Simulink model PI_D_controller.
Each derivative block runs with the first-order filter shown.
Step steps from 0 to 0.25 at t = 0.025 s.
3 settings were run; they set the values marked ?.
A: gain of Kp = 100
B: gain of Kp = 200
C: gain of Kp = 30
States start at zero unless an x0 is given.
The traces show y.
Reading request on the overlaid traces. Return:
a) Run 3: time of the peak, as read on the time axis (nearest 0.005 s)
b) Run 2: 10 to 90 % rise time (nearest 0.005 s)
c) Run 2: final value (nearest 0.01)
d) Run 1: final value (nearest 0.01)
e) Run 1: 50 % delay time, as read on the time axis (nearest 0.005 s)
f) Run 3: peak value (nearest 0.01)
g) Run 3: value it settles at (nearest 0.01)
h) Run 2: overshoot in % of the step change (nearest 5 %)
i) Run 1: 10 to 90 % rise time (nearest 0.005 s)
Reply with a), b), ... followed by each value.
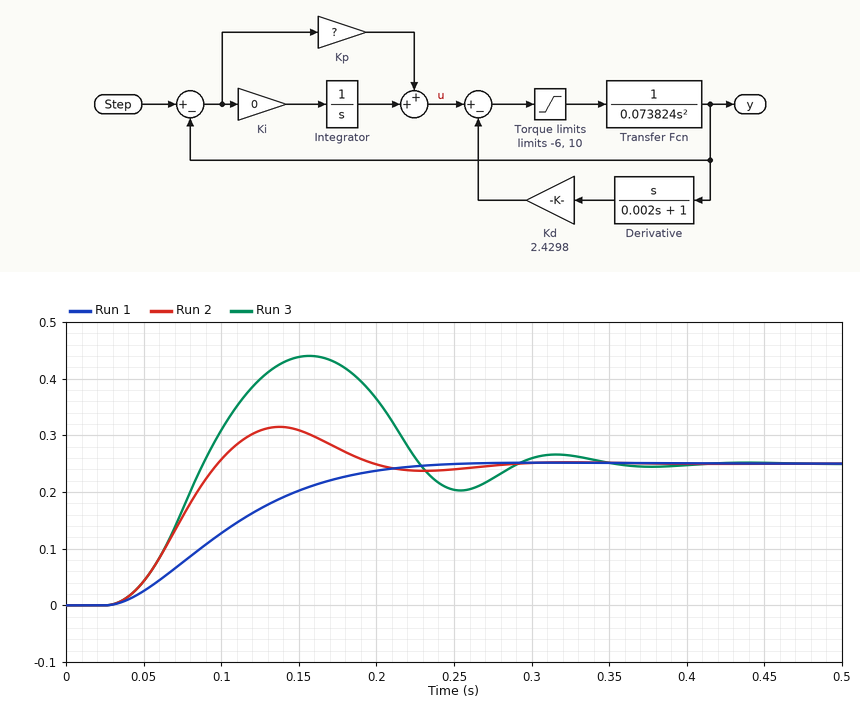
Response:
a) 0.155 s
b) 0.045 s
c) 0.25
d) 0.25
e) 0.100 s
f) 0.44
g) 0.25
h) 25 %
i) 0.125 s
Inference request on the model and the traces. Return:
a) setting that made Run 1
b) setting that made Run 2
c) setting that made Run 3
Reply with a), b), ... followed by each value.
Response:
a) C
b) A
c) B
